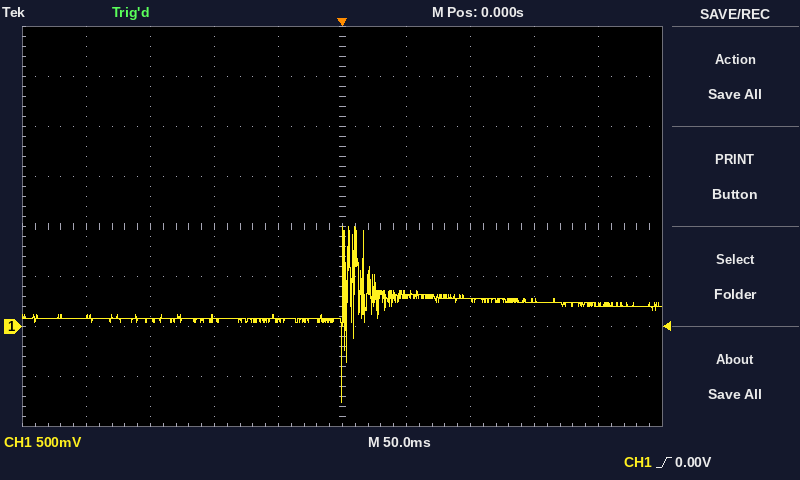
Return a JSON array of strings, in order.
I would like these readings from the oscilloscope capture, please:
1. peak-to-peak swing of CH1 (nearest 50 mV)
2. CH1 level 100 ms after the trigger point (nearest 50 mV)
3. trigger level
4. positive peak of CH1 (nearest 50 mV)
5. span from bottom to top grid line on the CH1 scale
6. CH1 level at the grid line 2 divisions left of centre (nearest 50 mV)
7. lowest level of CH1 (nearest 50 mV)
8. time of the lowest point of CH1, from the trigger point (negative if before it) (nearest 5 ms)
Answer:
["1.75 V", "250 mV", "0.00 V", "1.00 V", "4 V", "100 mV", "-750 mV", "0 ms"]
